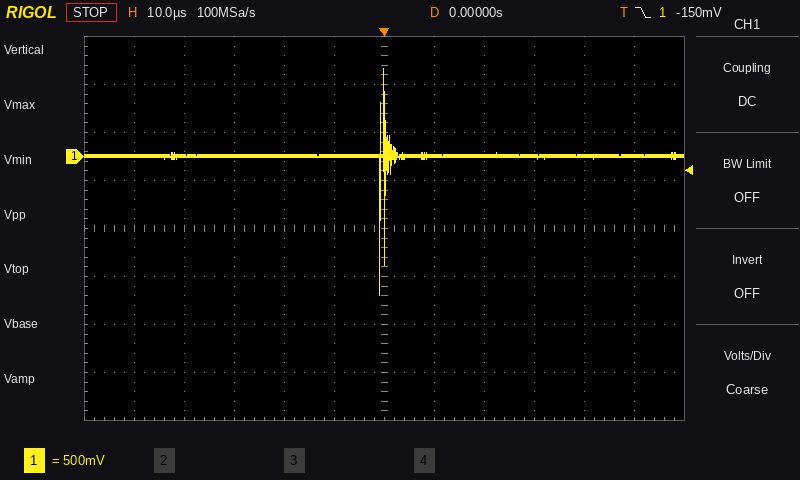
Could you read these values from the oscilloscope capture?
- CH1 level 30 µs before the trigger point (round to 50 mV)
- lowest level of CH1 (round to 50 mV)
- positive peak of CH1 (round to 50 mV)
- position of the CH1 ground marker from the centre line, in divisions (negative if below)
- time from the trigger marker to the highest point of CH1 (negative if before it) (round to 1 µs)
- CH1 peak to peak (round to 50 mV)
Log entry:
0 mV
-1.45 V
900 mV
+1.5 div
0 µs
2.35 V
